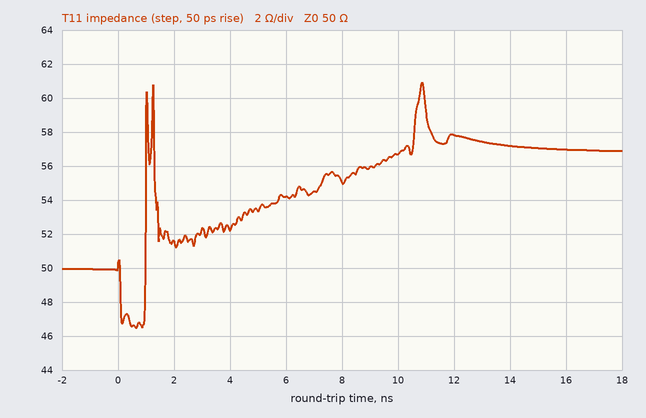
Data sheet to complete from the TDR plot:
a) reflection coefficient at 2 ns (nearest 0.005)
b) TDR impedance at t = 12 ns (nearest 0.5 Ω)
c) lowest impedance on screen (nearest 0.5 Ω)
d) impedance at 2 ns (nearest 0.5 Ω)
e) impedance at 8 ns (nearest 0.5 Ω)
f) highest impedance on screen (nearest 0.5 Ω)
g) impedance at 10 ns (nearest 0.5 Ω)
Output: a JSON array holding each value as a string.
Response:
["+0.015", "58.0 Ω", "46.5 Ω", "51.5 Ω", "55.0 Ω", "61.0 Ω", "56.5 Ω"]
